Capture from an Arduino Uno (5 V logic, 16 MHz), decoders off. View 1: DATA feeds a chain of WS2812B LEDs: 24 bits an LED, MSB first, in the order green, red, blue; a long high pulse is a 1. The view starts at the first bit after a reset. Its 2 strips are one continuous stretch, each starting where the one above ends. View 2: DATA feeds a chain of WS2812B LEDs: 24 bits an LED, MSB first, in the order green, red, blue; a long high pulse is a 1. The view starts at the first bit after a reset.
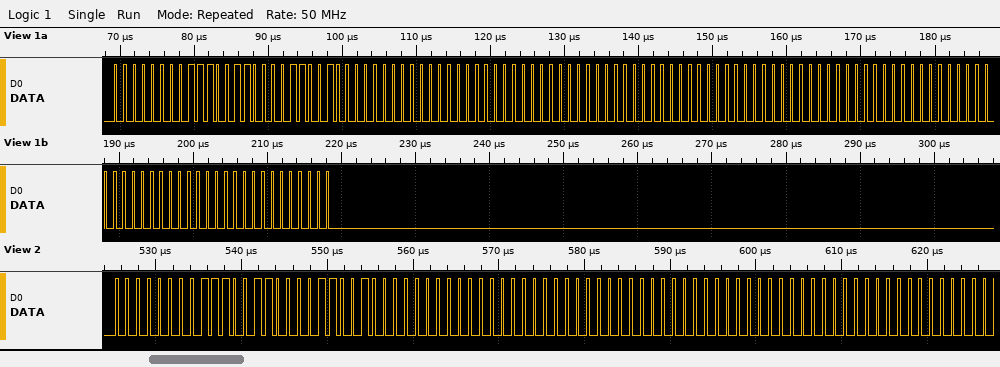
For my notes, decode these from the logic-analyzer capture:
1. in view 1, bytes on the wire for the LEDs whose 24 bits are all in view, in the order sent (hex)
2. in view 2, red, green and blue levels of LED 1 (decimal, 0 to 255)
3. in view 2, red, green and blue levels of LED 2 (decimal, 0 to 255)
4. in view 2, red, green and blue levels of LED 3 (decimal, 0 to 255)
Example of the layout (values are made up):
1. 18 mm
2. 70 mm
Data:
1. 00 E6 19 00 00 00 00 00 00 00 00 00 00 00 00
2. 230, 0, 25
3. 0, 0, 0
4. 0, 0, 0
